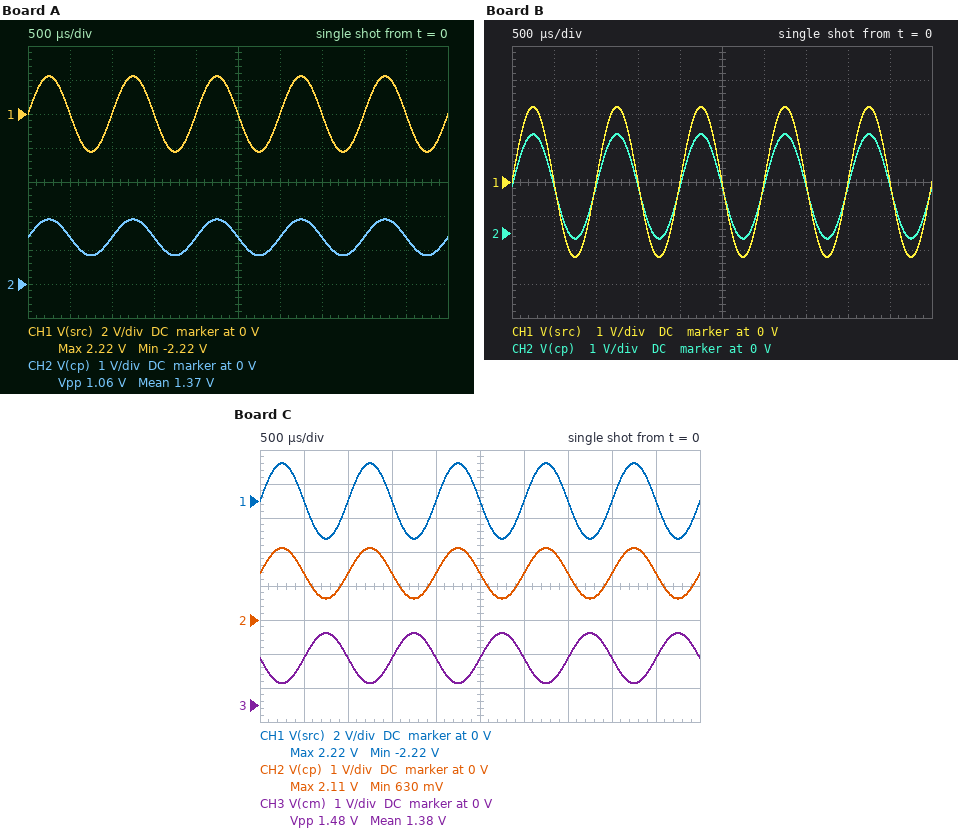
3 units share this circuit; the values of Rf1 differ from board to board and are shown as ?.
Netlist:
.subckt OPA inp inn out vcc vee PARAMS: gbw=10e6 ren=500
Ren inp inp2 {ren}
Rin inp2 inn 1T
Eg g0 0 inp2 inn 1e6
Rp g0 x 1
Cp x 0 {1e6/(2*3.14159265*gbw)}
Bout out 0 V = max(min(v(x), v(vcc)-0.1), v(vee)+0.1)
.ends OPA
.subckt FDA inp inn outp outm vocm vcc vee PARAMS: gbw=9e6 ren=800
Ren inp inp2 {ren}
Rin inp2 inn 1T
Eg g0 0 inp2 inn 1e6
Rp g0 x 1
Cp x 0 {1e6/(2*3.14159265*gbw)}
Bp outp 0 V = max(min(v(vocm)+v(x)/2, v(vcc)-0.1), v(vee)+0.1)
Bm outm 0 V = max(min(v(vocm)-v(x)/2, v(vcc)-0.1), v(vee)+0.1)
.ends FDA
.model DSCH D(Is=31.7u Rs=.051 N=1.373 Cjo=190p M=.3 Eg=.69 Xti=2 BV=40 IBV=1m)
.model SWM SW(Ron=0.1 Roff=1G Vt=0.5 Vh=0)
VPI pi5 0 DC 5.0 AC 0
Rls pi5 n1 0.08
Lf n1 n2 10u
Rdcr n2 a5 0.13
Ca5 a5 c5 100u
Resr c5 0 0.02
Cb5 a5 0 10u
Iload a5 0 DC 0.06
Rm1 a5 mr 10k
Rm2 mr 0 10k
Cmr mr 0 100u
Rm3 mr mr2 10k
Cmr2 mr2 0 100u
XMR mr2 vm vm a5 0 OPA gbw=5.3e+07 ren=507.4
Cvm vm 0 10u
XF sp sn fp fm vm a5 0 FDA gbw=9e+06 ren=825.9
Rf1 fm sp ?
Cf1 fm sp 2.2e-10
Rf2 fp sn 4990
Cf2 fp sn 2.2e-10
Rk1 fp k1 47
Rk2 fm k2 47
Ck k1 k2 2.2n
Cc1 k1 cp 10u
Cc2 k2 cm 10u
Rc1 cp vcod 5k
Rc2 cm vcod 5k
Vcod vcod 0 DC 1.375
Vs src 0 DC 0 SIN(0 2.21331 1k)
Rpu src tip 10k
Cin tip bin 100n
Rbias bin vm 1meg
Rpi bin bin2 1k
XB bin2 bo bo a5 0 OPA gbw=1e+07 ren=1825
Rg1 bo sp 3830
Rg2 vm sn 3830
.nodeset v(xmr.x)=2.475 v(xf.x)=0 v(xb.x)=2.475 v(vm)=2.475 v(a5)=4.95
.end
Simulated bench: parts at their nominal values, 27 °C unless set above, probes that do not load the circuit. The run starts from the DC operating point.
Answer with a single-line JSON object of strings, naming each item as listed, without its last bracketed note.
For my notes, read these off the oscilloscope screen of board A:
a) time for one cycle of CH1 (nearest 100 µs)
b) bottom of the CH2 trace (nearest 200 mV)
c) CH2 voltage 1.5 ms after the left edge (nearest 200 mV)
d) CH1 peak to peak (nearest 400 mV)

{"time for one cycle of CH1": "1.0 ms", "bottom of the CH2 trace": "800 mV", "CH2 voltage 1.5 ms after the left edge": "1.4 V", "CH1 peak to peak": "4.4 V"}
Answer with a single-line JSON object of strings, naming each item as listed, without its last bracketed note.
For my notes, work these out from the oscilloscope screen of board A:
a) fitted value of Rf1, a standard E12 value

{"fitted value of Rf1, a standard E12 value": "1.5 kΩ"}
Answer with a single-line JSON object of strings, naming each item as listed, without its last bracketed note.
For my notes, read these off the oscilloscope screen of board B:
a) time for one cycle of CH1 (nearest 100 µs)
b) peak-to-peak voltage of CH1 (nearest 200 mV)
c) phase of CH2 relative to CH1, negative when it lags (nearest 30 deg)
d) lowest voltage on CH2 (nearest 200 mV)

{"time for one cycle of CH1": "1.0 ms", "peak-to-peak voltage of CH1": "4.4 V", "phase of CH2 relative to CH1, negative when it lags": "0 deg", "lowest voltage on CH2": "-200 mV"}
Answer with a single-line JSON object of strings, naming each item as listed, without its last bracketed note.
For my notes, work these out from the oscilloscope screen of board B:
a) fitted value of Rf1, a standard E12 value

{"fitted value of Rf1, a standard E12 value": "5.6 kΩ"}
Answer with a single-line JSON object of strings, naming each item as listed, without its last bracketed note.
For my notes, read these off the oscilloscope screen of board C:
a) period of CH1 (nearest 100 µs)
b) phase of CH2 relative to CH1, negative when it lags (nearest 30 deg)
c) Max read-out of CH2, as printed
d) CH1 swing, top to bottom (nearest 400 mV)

{"period of CH1": "1.0 ms", "phase of CH2 relative to CH1, negative when it lags": "0 deg", "Max read-out of CH2, as printed": "2.11 V", "CH1 swing, top to bottom": "4.4 V"}
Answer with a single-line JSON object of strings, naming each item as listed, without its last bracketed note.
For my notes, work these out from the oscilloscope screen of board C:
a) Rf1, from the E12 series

{"Rf1, from the E12 series": "2.2 kΩ"}
